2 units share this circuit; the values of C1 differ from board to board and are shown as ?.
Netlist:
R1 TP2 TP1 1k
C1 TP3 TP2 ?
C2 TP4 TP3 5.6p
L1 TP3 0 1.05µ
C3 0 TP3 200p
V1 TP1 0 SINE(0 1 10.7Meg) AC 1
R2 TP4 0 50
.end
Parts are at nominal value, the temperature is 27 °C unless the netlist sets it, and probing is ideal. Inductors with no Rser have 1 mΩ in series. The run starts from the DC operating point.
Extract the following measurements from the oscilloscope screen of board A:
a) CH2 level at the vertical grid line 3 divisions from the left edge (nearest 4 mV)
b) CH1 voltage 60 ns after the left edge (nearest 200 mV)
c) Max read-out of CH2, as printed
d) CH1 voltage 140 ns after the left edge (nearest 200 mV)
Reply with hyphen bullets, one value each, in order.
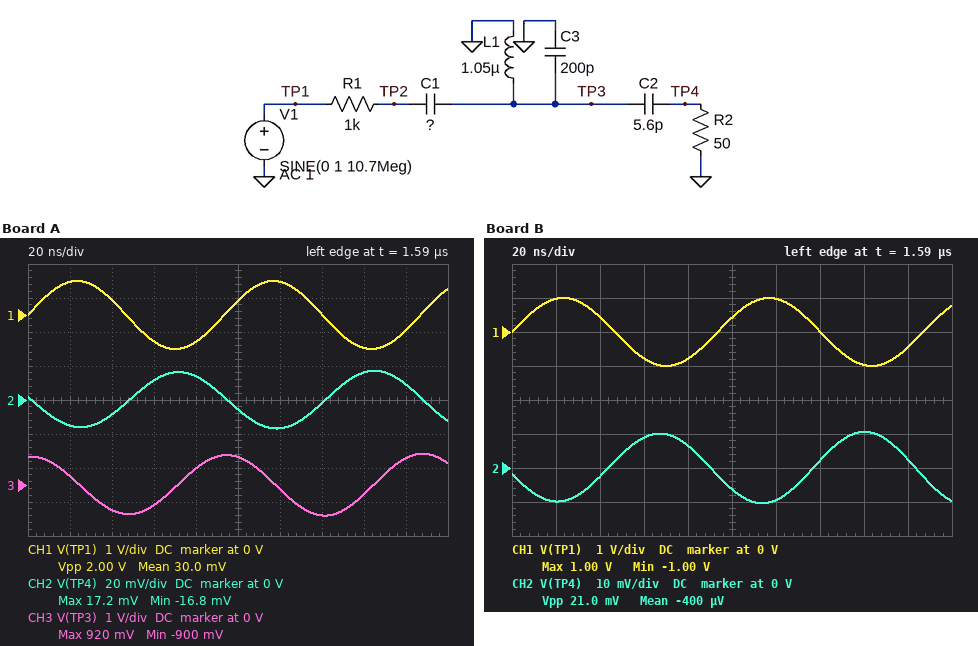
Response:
- 12 mV
- -800 mV
- 17.2 mV
- 0 V
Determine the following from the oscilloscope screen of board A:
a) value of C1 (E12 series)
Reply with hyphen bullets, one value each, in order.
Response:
- 3.9 pF
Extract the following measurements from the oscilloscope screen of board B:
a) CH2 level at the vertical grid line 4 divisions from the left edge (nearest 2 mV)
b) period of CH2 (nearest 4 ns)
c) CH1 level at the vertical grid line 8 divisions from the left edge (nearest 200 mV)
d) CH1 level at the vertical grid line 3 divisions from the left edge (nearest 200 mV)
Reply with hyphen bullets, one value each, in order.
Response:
- 6 mV
- 92 ns
- -1.0 V
- -800 mV
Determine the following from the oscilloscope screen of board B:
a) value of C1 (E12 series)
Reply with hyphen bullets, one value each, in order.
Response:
- 2.2 pF
